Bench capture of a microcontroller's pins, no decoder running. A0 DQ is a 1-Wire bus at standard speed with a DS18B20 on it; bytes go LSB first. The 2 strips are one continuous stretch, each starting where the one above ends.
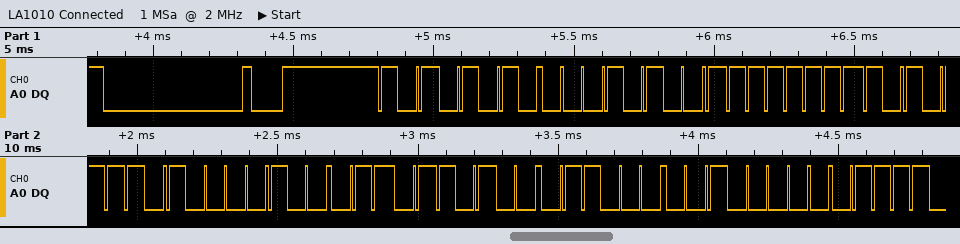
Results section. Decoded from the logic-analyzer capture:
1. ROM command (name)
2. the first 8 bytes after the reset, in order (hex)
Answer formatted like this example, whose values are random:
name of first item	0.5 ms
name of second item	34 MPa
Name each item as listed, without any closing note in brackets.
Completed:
ROM command	Match ROM
the first 8 bytes after the reset, in order	55 28 FF 75 21 B6 18 04
